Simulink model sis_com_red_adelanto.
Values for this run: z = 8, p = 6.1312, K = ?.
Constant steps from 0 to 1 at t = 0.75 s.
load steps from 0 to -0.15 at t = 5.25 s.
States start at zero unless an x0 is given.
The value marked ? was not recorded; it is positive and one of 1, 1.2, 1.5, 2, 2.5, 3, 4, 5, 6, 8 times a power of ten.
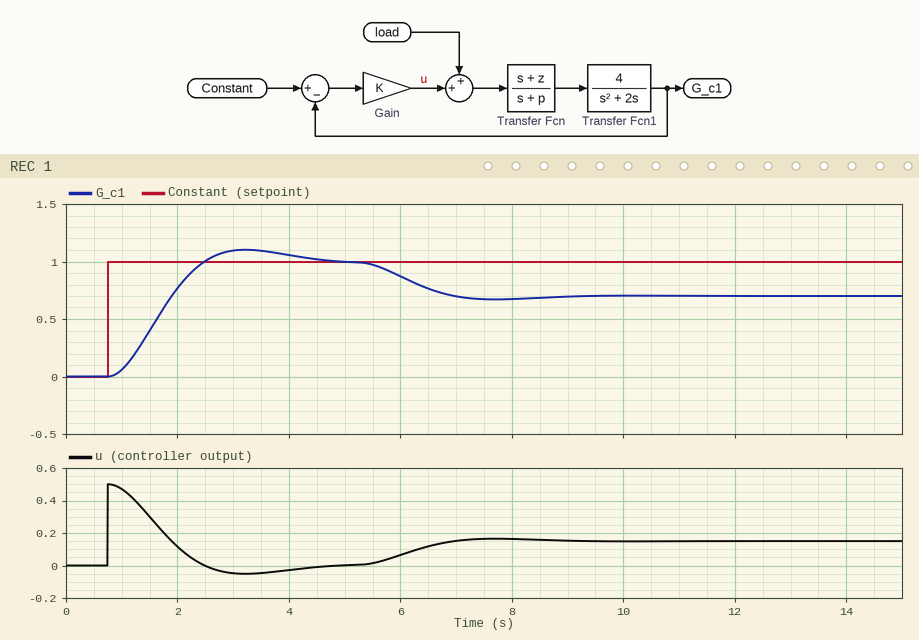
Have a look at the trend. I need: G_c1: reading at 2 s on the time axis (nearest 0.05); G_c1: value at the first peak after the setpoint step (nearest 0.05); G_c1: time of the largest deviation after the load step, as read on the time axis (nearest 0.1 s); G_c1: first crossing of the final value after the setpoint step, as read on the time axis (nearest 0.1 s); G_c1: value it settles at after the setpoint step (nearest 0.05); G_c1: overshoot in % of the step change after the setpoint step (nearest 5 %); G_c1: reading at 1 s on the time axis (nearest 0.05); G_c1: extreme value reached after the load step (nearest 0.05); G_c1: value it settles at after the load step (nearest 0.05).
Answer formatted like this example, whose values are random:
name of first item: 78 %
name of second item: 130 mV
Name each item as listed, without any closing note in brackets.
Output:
G_c1: reading at 2 s on the time axis: 0.75
G_c1: value at the first peak after the setpoint step: 1.10
G_c1: time of the largest deviation after the load step, as read on the time axis: 7.7 s
G_c1: first crossing of the final value after the setpoint step, as read on the time axis: 2.5 s
G_c1: value it settles at after the setpoint step: 1.00
G_c1: overshoot in % of the step change after the setpoint step: 10 %
G_c1: reading at 1 s on the time axis: 0.05
G_c1: extreme value reached after the load step: 0.65
G_c1: value it settles at after the load step: 0.70
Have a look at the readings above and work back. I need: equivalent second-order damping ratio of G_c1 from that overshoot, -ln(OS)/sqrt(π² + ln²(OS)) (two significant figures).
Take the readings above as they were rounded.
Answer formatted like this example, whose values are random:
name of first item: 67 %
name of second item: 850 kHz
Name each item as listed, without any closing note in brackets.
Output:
equivalent second-order damping ratio of G_c1 from that overshoot, -ln(OS)/sqrt(π² + ln²(OS)): 0.59
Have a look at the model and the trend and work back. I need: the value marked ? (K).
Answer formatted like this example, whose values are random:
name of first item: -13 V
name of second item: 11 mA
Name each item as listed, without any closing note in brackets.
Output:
the value marked ?: 0.5
